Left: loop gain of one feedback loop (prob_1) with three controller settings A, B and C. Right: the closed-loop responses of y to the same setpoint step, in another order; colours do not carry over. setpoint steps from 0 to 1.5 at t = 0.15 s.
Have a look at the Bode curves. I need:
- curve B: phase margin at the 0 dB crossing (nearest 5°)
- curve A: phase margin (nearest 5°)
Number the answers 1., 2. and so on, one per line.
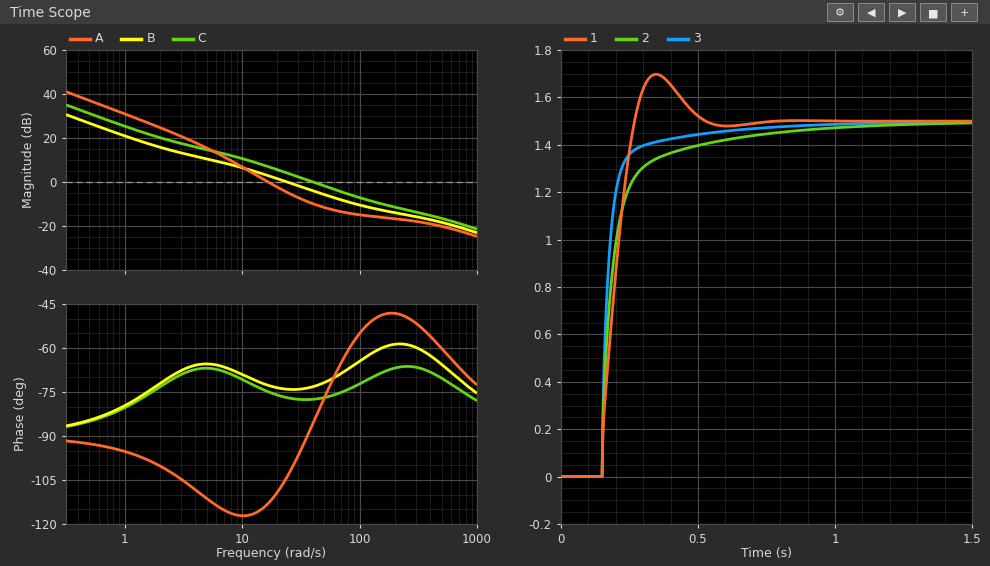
1. 105°
2. 65°
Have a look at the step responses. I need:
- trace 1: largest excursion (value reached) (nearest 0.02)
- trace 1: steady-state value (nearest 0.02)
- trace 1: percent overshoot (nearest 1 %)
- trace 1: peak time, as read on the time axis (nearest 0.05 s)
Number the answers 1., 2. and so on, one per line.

1. 1.70
2. 1.50
3. 13 %
4. 0.35 s
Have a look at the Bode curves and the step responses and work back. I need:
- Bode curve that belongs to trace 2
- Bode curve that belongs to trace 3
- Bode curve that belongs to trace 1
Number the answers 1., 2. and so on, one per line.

1. B
2. C
3. A
